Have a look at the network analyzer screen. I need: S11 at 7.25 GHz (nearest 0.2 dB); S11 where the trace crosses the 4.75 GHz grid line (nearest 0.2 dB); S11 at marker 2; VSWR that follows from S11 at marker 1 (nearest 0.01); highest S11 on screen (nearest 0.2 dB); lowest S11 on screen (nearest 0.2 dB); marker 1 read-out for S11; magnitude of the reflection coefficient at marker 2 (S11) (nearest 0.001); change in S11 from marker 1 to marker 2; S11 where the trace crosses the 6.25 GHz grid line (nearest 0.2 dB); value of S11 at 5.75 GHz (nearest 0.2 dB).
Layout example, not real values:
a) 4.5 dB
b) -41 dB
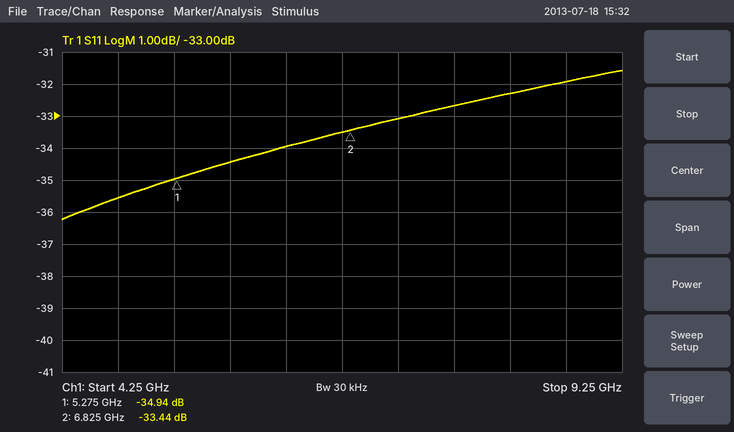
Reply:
a) -33.0 dB
b) -35.6 dB
c) -33.44 dB
d) 1.04
e) -31.6 dB
f) -36.2 dB
g) -34.94 dB
h) 0.021
i) 1.50 dB
j) -34.0 dB
k) -34.4 dB
